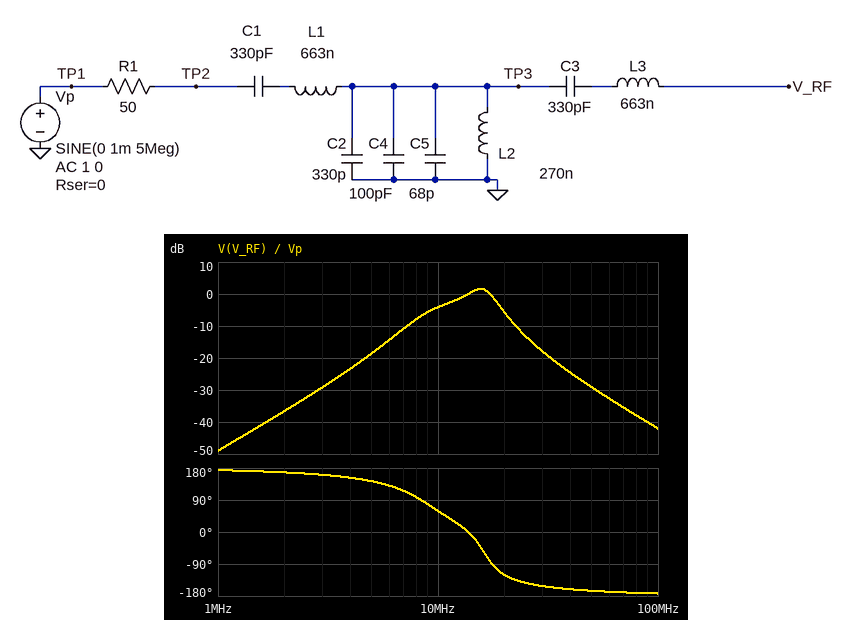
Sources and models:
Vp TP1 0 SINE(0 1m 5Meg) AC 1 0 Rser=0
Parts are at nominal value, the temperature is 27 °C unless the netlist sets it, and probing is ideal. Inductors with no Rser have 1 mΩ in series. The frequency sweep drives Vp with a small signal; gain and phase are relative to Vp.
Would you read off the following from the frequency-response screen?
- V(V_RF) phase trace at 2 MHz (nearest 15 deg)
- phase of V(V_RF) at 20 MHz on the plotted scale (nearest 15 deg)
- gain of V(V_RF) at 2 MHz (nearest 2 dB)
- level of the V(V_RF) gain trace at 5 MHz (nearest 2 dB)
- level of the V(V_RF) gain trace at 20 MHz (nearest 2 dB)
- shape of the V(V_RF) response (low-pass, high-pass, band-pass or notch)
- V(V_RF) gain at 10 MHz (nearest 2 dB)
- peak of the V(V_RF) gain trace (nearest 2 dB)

165 deg
-120 deg
-36 dB
-18 dB
-6 dB
band-pass
-4 dB
2 dB
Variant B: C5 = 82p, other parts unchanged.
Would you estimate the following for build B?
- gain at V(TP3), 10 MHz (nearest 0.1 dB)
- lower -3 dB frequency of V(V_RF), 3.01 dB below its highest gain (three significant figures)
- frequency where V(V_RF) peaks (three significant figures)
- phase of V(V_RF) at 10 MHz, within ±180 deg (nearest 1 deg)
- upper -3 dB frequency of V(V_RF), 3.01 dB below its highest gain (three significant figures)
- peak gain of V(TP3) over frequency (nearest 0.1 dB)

-3.9 dB
12.2 MHz
15.4 MHz
58 deg
17.7 MHz
1.5 dB
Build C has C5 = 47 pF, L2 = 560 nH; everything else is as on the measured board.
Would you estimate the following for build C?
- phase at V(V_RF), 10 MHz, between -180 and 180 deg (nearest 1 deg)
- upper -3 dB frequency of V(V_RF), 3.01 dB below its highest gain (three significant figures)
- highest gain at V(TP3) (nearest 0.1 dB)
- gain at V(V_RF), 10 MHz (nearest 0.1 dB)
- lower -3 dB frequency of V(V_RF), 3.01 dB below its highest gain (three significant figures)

-4 deg
14.7 MHz
0.9 dB
-0.1 dB
6.42 MHz
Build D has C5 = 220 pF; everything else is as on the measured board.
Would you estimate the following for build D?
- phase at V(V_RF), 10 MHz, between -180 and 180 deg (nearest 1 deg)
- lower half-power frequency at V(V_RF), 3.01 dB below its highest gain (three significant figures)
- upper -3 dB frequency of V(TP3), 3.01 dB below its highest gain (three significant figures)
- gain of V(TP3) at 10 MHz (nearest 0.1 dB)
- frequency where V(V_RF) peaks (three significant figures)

46 deg
9.64 MHz
15.7 MHz
-2.0 dB
13.1 MHz
